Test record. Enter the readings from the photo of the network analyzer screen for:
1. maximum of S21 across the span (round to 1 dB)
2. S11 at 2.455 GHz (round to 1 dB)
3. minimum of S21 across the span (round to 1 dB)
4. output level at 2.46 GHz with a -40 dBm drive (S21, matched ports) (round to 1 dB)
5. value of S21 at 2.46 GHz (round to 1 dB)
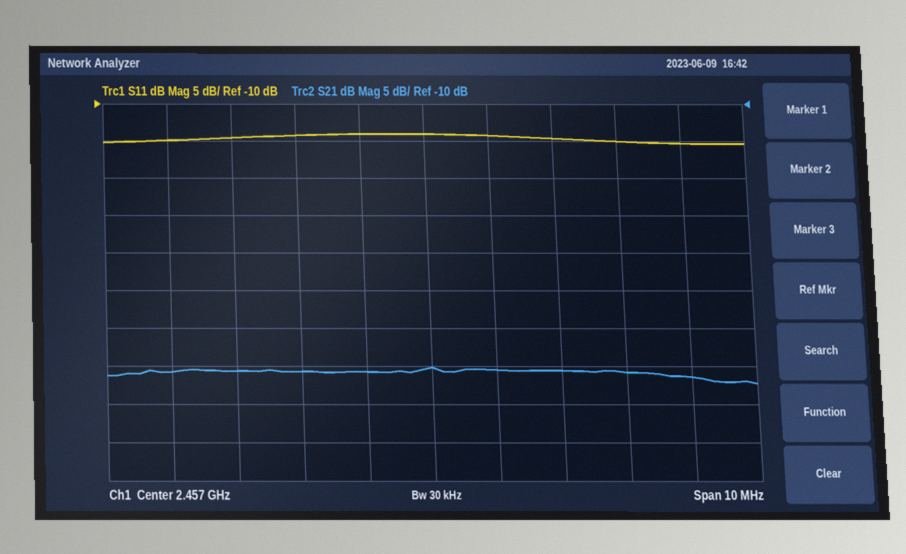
-45 dB
-14 dB
-47 dB
-86 dBm
-46 dB
